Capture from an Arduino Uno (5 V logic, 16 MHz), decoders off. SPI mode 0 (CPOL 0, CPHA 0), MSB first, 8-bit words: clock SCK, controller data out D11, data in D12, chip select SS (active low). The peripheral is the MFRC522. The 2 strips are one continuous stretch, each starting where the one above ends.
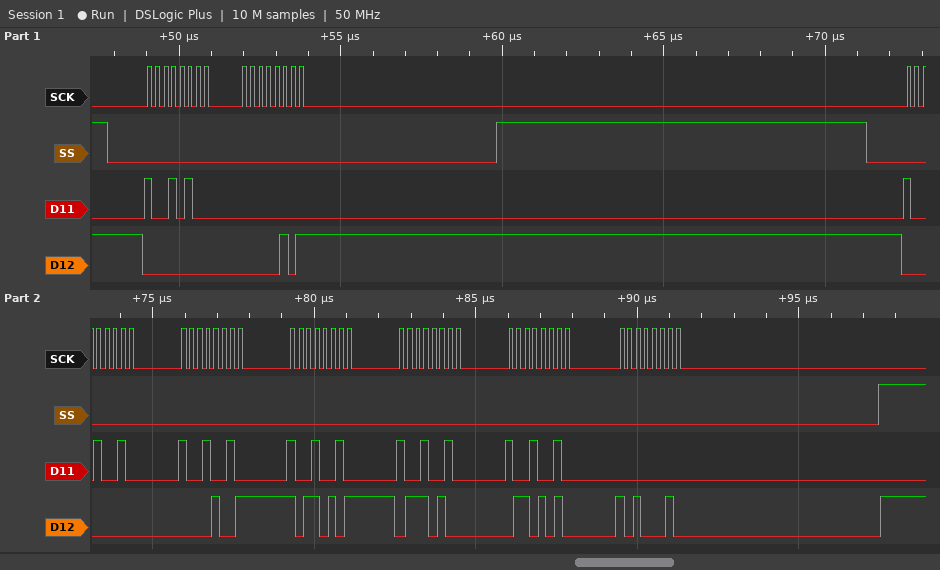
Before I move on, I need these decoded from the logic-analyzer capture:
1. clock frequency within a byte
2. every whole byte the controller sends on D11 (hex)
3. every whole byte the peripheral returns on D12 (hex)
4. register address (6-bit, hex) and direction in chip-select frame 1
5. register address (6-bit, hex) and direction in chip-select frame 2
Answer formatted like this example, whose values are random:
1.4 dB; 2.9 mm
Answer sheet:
4 MHz; 94 00 92 92 92 92 92 00; 00 05 00 09 B5 74 6A A2; 0x0A read; 0x09 read
